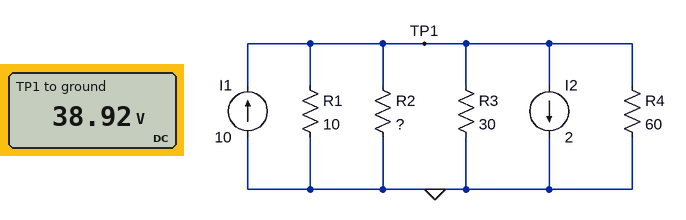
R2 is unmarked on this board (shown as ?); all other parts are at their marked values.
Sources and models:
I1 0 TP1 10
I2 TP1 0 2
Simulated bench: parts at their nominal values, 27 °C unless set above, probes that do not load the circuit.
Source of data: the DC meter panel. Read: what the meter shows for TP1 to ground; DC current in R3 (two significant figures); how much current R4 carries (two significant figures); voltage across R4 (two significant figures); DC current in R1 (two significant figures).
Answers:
38.92 V
1.3 A
650 mA
39 V
3.9 A
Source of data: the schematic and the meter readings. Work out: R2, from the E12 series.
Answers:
18 Ω
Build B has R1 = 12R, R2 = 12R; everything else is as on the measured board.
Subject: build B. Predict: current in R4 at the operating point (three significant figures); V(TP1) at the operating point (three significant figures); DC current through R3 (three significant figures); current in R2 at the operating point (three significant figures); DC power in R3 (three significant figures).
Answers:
615 mA
36.9 V
1.23 A
3.08 A
45.4 W
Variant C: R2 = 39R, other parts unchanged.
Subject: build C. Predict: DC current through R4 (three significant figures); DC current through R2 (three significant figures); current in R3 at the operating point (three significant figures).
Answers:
759 mA
1.17 A
1.52 A
